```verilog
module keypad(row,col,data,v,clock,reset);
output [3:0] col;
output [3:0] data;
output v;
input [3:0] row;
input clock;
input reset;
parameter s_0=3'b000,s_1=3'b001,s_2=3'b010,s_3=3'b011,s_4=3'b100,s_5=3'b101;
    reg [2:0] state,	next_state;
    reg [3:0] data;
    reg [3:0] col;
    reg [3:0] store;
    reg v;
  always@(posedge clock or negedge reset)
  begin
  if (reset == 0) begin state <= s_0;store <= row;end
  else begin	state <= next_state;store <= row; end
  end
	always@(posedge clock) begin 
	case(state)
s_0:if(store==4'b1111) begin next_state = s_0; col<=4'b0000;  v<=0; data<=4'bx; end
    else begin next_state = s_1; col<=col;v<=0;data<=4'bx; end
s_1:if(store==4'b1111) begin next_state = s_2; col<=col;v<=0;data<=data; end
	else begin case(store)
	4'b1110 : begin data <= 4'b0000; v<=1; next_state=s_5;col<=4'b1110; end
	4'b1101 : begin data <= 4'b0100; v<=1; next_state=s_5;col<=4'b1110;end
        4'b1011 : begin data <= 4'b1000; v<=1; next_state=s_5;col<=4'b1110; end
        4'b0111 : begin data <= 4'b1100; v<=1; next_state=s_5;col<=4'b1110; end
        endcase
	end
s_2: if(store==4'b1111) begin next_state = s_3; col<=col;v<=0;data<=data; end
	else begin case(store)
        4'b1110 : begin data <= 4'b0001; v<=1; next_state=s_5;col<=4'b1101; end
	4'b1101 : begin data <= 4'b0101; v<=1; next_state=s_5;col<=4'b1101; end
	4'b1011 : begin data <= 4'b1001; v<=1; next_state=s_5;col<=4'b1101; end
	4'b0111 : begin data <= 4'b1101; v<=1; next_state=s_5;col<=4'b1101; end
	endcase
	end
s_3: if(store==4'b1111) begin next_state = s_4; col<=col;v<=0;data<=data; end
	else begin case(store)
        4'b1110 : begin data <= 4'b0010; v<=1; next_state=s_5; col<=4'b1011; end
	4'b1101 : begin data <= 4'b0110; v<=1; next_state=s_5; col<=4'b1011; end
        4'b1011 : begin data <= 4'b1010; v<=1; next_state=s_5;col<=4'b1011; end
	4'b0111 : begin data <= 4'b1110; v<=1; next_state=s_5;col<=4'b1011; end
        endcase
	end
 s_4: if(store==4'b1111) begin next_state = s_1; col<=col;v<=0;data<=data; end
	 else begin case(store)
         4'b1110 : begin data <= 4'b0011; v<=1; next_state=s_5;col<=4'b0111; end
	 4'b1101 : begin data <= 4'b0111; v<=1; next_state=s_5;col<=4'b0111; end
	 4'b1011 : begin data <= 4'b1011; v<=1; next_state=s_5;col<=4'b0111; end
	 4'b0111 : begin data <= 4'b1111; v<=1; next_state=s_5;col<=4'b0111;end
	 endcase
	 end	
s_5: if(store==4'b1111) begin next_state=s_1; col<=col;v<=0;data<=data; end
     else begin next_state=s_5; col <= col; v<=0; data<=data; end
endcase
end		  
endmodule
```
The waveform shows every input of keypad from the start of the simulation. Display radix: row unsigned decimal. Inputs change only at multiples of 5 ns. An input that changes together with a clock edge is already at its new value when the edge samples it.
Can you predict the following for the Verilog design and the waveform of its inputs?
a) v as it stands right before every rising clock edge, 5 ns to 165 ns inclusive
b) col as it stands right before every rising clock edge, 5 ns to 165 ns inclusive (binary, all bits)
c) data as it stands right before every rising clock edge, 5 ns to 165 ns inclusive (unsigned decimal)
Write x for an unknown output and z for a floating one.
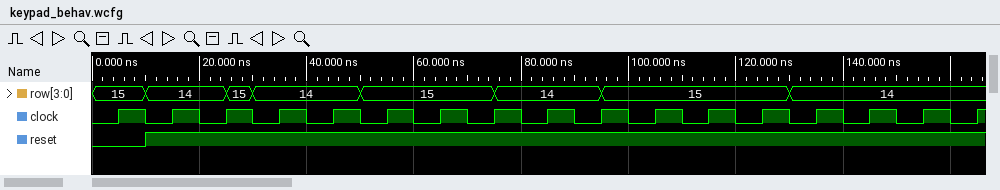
x 0 0 0 0 1 0 0 0 1 1 0 0 0 0 1 1
x, 0000, 0000, 0000, 0000, 1110, 1110, 1110, 1110, 1110, 1101, 1101, 1101, 1101, 1101, 1101, 1101
x, x, x, x, x, 0, x, x, x, 0, 1, 1, 1, 1, 1, 1, 1
